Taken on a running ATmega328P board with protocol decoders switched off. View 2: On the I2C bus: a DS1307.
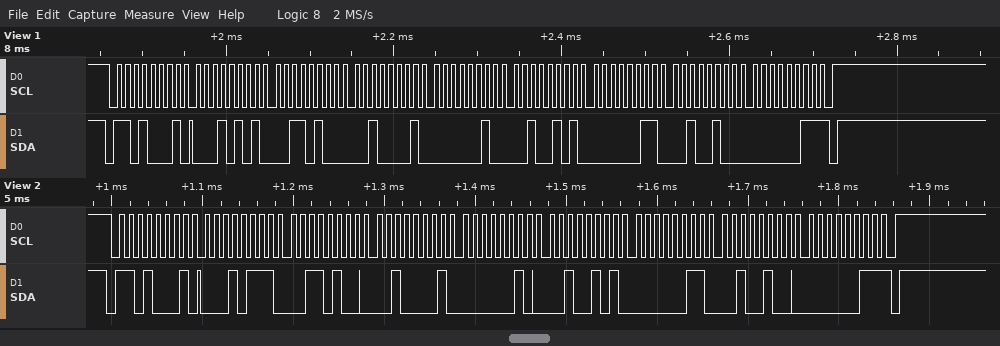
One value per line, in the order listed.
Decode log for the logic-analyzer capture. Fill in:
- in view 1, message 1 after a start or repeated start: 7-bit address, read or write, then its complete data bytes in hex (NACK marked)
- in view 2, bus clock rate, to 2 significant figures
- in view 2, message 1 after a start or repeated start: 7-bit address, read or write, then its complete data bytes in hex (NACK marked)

0x68 read: 15 34 21 02 25 03 24 03 NACK
100 kHz
0x68 read: 17 34 21 02 25 03 24 03 NACK
